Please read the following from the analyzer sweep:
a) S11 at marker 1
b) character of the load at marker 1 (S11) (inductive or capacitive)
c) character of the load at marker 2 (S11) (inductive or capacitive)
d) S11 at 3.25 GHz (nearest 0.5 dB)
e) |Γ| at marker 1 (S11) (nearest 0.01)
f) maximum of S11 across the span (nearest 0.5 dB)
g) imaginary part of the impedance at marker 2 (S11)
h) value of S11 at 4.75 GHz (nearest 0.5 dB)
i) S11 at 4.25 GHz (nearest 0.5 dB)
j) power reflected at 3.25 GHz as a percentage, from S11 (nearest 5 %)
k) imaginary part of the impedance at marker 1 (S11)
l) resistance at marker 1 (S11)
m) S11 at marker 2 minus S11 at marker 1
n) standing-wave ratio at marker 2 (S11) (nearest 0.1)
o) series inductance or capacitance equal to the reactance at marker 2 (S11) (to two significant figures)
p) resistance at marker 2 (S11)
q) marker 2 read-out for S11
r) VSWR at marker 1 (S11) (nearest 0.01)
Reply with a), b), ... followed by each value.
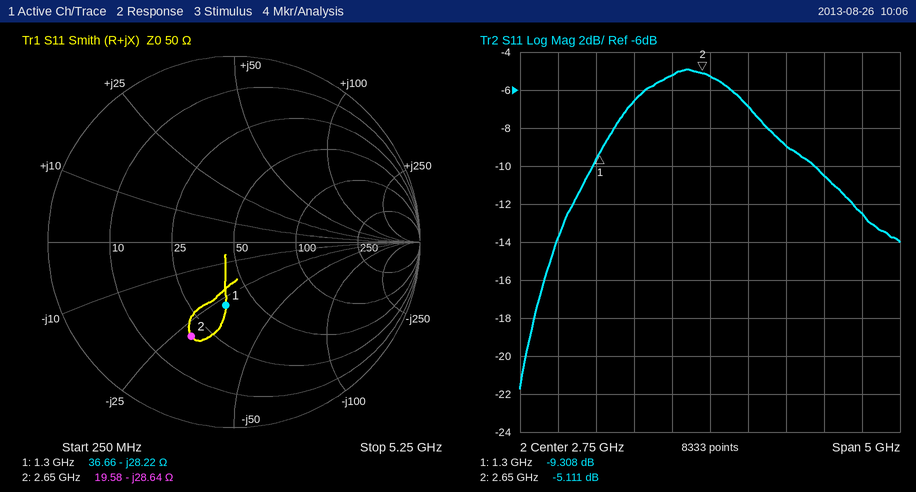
a) -9.308 dB
b) capacitive
c) capacitive
d) -7.0 dB
e) 0.34
f) -5.0 dB
g) -28.64 Ω
h) -12.5 dB
i) -10.5 dB
j) 20 %
k) -28.22 Ω
l) 36.66 Ω
m) 4.197 dB
n) 3.5
o) 2.1 pF
p) 19.58 Ω
q) -5.111 dB
r) 2.04
